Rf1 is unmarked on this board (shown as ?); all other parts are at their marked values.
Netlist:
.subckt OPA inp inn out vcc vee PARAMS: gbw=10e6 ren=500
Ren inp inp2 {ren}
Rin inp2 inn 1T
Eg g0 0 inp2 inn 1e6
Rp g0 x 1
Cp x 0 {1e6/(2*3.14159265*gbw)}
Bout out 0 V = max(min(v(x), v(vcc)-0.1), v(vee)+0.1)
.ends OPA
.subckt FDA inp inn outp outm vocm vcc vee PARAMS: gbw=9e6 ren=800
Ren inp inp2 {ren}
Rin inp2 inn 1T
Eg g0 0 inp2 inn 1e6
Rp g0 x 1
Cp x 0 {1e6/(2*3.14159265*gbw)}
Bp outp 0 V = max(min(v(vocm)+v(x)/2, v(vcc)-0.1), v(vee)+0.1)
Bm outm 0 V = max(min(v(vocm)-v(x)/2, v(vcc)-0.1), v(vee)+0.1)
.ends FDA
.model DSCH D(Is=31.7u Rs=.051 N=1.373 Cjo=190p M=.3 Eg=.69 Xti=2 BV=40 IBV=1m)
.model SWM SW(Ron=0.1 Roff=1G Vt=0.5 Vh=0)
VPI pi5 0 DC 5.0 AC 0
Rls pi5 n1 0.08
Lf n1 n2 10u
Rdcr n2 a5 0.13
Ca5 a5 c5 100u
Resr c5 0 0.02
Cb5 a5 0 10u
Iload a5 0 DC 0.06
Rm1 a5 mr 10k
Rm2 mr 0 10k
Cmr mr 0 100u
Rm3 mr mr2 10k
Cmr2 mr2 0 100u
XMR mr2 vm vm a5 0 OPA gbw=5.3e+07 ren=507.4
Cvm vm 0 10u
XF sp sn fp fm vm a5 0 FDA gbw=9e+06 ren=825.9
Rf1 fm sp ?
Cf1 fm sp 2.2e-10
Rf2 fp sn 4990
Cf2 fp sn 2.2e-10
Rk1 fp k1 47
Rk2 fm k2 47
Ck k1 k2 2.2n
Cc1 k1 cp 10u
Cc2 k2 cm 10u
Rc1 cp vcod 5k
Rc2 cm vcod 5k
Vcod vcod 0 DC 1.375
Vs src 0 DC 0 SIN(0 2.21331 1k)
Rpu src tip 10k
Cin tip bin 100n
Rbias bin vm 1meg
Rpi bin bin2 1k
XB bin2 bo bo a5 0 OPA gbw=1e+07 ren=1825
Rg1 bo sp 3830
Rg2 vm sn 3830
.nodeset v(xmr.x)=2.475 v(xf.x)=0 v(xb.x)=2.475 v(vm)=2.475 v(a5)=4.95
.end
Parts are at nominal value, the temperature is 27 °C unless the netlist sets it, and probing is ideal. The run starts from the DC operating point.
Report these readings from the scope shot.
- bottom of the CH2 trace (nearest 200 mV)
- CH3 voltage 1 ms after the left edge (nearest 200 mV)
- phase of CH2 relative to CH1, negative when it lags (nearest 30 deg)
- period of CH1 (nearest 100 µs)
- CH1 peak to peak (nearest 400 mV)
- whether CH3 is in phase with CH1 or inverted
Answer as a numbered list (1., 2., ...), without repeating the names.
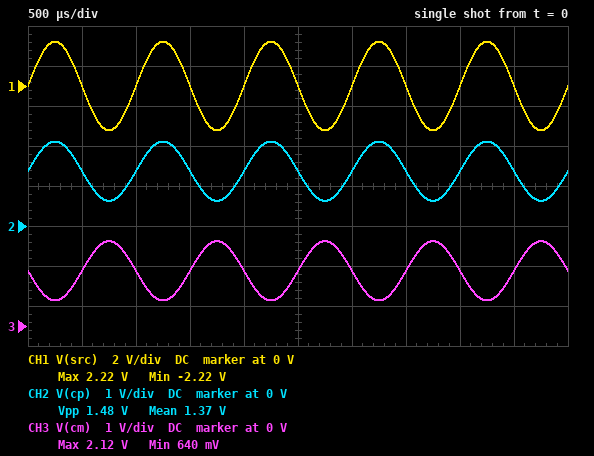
1. 600 mV
2. 1.4 V
3. 0 deg
4. 1.0 ms
5. 4.4 V
6. inverted
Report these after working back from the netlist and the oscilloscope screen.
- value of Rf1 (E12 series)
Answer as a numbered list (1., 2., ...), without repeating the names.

1. 2.2 kΩ
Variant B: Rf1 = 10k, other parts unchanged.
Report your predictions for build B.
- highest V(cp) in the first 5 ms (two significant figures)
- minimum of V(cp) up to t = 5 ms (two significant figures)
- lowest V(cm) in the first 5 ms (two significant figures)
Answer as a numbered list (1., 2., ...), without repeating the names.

1. 3.6 V
2. -840 mV
3. -820 mV
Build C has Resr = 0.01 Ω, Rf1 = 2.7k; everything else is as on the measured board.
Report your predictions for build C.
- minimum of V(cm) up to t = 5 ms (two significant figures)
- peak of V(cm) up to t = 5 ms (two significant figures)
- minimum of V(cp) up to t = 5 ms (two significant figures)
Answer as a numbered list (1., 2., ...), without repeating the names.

1. 500 mV
2. 2.3 V
3. 490 mV
